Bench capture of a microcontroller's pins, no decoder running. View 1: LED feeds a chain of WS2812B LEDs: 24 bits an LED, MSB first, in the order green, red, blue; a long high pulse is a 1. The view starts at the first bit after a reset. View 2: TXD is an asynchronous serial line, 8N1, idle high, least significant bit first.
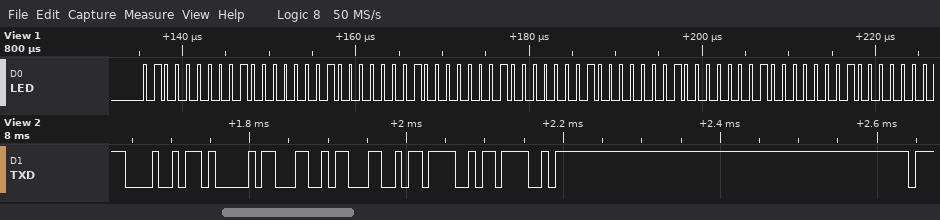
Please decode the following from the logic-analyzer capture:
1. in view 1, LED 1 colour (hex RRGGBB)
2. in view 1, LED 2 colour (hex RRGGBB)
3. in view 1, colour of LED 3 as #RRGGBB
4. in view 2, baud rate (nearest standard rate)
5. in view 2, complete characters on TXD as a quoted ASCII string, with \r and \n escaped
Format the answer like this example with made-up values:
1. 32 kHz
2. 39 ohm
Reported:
1. #404040
2. #404040
3. #404040
4. 115200 baud
5. "HALLOO"
